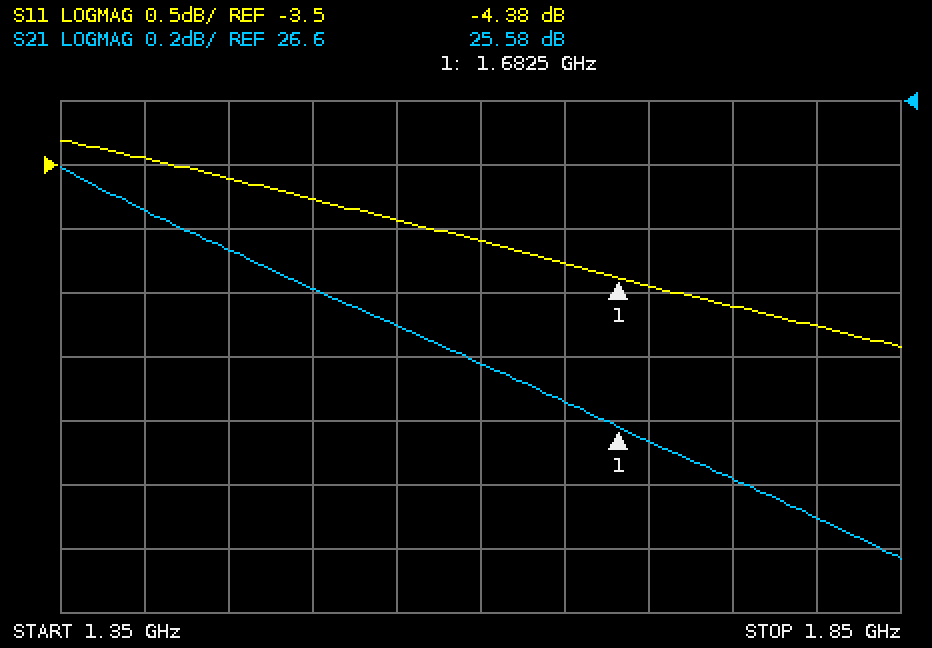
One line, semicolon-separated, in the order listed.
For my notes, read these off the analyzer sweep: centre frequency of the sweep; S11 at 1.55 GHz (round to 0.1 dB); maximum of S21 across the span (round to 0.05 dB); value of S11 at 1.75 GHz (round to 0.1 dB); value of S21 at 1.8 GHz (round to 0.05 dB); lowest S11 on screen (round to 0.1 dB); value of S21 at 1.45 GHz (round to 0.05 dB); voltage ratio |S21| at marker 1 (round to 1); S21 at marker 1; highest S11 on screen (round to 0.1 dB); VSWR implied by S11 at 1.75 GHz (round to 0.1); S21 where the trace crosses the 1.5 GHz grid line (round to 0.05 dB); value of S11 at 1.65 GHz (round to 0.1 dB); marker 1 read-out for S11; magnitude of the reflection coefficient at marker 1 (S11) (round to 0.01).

1.6 GHz; -3.9 dB; 26.40 dB; -4.6 dB; 25.30 dB; -4.9 dB; 26.15 dB; 19; 25.58 dB; -3.3 dB; 3.9; 26.00 dB; -4.3 dB; -4.38 dB; 0.60
